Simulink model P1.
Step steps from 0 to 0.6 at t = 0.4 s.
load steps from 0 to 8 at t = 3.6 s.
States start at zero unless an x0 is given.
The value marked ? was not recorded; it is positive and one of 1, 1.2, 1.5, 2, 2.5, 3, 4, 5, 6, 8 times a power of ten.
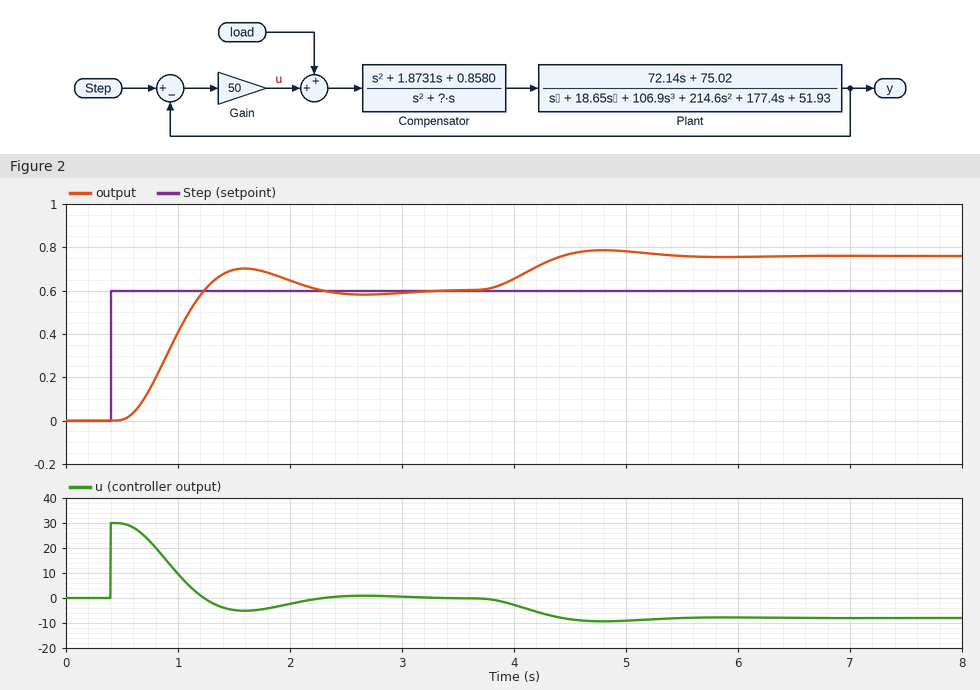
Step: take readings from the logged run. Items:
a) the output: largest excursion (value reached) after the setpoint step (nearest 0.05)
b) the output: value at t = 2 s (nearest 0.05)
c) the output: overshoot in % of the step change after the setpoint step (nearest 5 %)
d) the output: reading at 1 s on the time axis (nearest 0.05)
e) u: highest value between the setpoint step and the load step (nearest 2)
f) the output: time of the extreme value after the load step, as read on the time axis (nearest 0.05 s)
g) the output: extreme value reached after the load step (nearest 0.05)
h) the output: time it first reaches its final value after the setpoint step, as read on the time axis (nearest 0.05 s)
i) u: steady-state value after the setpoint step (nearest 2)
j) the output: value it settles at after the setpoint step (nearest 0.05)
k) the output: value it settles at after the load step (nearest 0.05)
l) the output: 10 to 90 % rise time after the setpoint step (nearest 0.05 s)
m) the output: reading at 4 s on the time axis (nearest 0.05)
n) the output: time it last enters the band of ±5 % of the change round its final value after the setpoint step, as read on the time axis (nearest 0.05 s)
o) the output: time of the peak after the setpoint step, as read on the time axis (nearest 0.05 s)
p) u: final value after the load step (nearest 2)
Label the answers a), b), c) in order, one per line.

a) 0.70
b) 0.65
c) 15 %
d) 0.40
e) 30
f) 4.80 s
g) 0.80
h) 1.25 s
i) 0
j) 0.60
k) 0.75
l) 0.50 s
m) 0.65
n) 2.10 s
o) 1.60 s
p) -8
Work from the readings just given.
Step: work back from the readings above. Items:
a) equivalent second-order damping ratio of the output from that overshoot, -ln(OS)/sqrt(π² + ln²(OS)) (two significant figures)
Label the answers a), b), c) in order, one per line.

a) 0.52
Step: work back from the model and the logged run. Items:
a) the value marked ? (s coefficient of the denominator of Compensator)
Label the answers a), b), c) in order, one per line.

a) 25
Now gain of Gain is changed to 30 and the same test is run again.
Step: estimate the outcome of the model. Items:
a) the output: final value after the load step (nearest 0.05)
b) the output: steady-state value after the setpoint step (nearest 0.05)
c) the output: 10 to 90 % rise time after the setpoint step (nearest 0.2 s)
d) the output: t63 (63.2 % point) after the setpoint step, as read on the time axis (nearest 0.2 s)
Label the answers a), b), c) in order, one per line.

a) 0.85
b) 0.60
c) 0.8 s
d) 1.2 s
